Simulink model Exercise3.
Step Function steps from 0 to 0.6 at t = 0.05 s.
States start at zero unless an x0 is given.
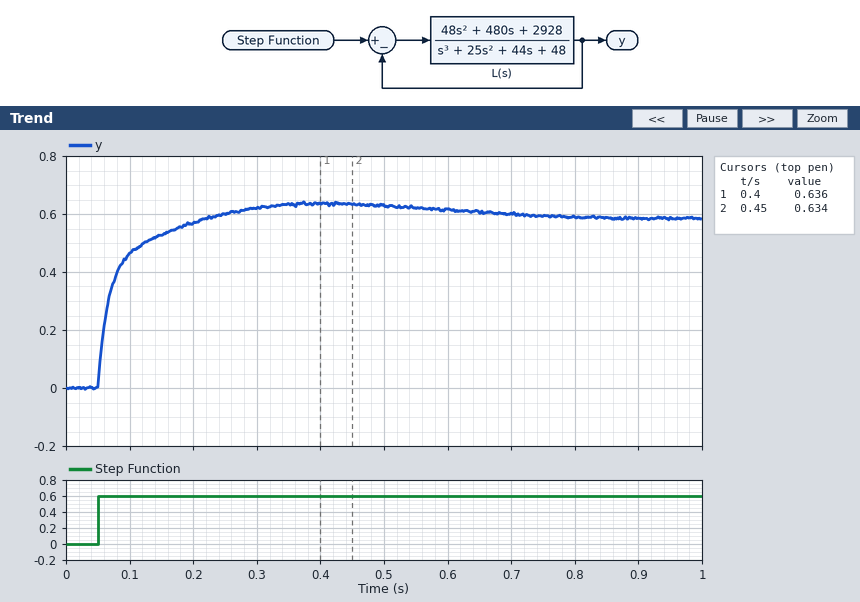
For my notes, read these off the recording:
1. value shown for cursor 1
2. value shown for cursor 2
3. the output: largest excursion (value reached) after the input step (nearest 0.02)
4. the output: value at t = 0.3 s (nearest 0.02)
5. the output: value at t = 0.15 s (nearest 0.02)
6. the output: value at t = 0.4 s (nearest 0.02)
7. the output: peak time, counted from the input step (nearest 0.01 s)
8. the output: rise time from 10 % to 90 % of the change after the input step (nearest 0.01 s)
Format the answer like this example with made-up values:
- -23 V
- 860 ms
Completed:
- 0.636
- 0.634
- 0.64
- 0.62
- 0.52
- 0.64
- 0.36 s
- 0.10 s
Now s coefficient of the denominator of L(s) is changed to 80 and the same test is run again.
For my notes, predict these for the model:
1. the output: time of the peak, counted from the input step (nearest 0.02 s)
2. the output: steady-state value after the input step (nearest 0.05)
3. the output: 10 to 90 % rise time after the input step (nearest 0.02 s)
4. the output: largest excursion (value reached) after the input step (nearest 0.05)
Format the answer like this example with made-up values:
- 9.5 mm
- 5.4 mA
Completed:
- 0.40 s
- 0.60
- 0.12 s
- 0.60
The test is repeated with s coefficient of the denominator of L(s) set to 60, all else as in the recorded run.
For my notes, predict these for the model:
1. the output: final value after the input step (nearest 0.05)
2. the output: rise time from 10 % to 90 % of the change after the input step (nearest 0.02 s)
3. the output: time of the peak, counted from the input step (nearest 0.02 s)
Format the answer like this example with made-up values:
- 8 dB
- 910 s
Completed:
- 0.60
- 0.10 s
- 0.38 s
